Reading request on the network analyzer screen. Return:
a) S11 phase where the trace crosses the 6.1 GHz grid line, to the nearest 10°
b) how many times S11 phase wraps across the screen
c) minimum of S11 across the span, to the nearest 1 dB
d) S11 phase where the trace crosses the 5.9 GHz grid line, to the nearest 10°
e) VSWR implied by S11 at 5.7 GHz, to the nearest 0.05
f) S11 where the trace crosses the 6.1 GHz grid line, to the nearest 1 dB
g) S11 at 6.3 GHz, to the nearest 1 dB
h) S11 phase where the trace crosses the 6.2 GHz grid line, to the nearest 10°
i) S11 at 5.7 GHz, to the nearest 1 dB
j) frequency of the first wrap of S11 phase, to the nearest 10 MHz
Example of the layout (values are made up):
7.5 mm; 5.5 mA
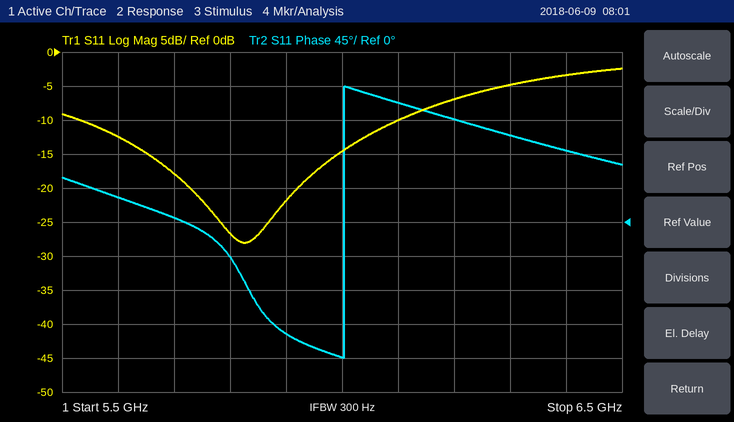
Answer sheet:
160°; 1; -28 dB; -150°; 1.30; -10 dB; -5 dB; 140°; -18 dB; 6.00 GHz
